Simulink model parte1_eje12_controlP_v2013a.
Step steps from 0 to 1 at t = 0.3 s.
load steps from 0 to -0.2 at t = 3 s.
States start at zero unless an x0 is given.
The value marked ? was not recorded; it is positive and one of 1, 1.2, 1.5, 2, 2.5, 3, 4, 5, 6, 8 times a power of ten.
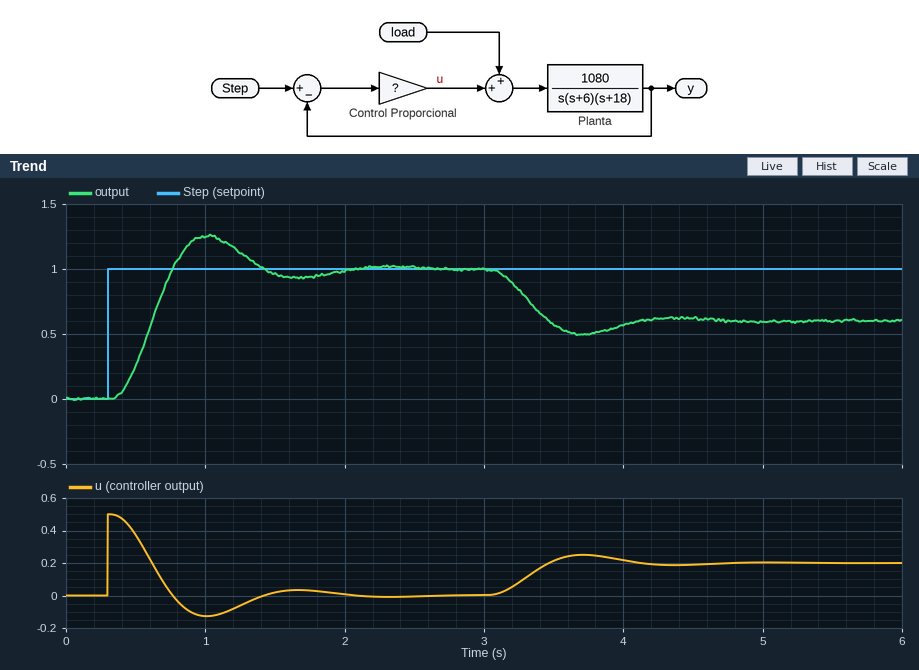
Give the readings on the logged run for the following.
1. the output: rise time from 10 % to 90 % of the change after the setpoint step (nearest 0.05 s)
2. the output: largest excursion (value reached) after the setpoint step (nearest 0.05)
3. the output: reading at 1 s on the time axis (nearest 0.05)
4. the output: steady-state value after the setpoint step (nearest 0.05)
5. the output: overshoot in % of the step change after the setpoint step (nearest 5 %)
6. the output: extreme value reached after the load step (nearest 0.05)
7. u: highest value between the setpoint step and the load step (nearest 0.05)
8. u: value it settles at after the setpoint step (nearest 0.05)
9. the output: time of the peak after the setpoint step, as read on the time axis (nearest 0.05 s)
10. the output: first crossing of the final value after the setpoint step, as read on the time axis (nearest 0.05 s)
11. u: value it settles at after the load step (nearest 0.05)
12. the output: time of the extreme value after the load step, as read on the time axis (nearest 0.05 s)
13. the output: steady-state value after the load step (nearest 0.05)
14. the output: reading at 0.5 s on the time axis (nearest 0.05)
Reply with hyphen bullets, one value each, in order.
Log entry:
- 0.30 s
- 1.25
- 1.25
- 1.00
- 25 %
- 0.50
- 0.50
- 0.00
- 1.00 s
- 0.75 s
- 0.20
- 3.70 s
- 0.60
- 0.25
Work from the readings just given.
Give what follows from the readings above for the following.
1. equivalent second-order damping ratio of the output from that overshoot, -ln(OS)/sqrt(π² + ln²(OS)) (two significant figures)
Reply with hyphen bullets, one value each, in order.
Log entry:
- 0.40
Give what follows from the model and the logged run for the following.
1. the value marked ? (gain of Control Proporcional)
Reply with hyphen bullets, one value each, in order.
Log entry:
- 0.5
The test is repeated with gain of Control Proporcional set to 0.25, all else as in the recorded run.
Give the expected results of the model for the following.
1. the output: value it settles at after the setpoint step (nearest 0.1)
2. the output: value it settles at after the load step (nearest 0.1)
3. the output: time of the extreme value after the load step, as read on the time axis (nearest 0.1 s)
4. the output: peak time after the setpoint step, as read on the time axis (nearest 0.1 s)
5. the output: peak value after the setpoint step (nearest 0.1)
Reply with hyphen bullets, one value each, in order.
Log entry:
- 1.0
- 0.2
- 4.2 s
- 1.5 s
- 1.1
